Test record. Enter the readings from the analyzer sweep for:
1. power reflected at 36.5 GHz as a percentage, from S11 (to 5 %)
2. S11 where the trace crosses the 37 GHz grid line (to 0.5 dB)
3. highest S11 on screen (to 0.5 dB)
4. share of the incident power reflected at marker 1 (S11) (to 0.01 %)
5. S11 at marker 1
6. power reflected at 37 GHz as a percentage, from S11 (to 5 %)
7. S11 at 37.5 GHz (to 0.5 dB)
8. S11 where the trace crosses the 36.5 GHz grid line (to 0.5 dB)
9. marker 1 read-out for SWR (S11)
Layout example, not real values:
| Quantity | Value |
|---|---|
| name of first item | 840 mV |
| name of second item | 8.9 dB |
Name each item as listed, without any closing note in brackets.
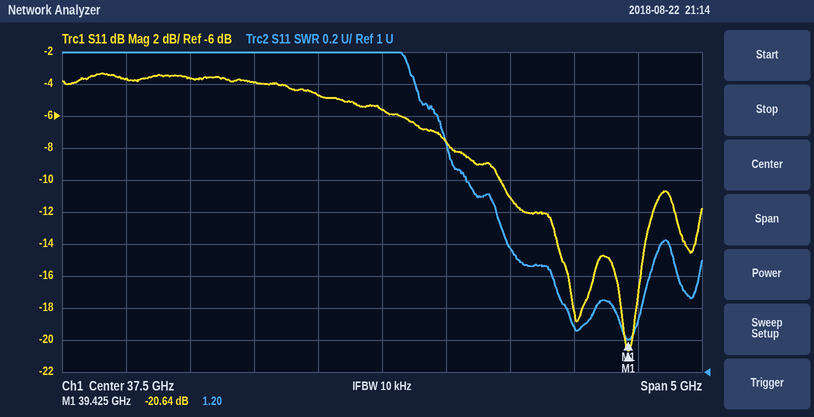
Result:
| Quantity | Value |
|---|---|
| power reflected at 36.5 GHz as a percentage, from S11 | 40 % |
| S11 where the trace crosses the 37 GHz grid line | -4.5 dB |
| highest S11 on screen | -3.5 dB |
| share of the incident power reflected at marker 1 (S11) | 0.86 % |
| S11 at marker 1 | -20.64 dB |
| power reflected at 37 GHz as a percentage, from S11 | 35 % |
| S11 at 37.5 GHz | -5.5 dB |
| S11 where the trace crosses the 36.5 GHz grid line | -4.0 dB |
| marker 1 read-out for SWR | 1.20 |
